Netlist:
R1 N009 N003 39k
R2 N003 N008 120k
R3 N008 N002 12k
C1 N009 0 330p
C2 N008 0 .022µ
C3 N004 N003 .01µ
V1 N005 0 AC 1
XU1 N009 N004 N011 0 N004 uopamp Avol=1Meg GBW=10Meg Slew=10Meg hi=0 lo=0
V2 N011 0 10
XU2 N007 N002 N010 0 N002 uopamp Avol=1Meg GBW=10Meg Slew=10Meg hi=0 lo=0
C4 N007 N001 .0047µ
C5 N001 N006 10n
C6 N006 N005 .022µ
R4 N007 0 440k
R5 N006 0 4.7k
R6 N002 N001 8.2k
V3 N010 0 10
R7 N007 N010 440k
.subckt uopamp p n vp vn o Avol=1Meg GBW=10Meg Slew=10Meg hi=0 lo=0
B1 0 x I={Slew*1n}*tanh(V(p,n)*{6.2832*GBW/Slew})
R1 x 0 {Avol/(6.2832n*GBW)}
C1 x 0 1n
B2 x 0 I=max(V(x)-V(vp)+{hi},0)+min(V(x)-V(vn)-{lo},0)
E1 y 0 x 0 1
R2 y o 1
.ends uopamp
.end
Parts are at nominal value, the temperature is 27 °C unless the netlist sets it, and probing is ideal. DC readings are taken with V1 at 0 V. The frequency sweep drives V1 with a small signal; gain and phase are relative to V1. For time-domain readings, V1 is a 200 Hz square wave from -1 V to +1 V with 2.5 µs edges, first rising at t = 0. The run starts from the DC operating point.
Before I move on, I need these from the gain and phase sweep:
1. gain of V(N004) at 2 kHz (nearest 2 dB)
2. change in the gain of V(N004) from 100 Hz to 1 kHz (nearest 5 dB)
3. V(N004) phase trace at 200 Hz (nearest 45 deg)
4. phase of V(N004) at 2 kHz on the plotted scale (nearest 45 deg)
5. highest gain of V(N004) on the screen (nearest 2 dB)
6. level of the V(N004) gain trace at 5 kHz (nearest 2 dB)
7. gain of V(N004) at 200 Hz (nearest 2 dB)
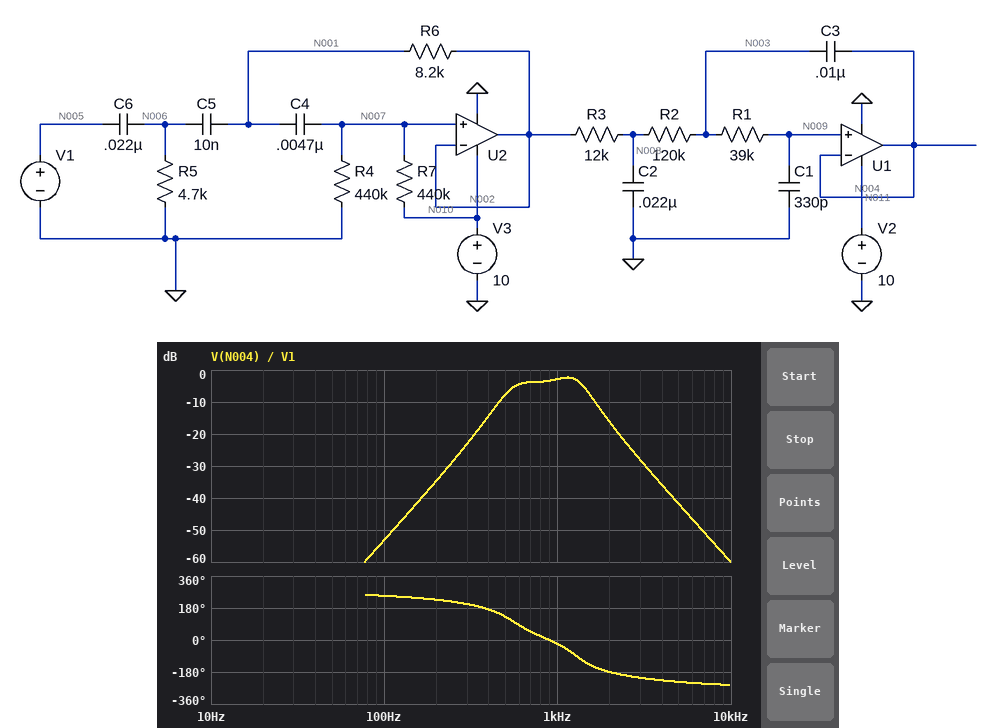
-16 dB
50 dB
225 deg
-180 deg
-2 dB
-42 dB
-34 dB
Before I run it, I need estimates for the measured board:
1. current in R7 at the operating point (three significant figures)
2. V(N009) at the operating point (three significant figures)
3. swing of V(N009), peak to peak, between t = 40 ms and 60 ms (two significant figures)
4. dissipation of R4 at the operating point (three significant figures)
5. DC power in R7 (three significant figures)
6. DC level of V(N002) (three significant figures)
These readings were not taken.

11.4 µA
5.00 V
1.1 V
56.8 µW
56.8 µW
5.00 V
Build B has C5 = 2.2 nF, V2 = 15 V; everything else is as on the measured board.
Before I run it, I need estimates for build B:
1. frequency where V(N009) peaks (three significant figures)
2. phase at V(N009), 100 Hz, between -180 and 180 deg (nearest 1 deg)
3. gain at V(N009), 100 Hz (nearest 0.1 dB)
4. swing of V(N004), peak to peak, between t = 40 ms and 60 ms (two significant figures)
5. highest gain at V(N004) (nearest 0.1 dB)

1.22 kHz
-108 deg
-66.4 dB
820 mV
2.5 dB
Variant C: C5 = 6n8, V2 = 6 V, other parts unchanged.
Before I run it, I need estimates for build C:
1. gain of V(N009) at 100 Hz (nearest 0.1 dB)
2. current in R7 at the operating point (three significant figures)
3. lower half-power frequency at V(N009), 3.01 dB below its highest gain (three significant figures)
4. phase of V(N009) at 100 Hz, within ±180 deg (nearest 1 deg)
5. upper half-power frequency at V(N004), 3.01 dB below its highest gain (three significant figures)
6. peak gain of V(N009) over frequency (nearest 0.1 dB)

-56.5 dB
11.4 µA
635 Hz
-110 deg
1.40 kHz
-1.3 dB
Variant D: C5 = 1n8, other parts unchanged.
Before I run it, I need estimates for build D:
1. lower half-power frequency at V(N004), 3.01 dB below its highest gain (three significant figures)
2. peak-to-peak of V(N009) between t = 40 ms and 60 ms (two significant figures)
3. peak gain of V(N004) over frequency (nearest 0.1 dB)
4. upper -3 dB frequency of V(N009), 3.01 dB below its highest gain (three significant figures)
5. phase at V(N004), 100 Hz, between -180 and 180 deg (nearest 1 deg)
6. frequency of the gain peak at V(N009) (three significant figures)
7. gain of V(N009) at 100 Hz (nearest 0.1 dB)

1.10 kHz
750 mV
1.6 dB
1.49 kHz
-107 deg
1.28 kHz
-68.2 dB
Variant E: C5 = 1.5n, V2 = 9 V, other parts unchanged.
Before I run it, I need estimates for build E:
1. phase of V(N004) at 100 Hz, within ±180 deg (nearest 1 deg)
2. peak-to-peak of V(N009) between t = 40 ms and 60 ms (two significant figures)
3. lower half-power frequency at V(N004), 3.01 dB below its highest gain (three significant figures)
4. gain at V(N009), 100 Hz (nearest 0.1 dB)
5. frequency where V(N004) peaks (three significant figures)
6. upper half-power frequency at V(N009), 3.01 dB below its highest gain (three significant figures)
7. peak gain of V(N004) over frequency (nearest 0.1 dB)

-107 deg
690 mV
1.13 kHz
-69.8 dB
1.33 kHz
1.56 kHz
0 dB
